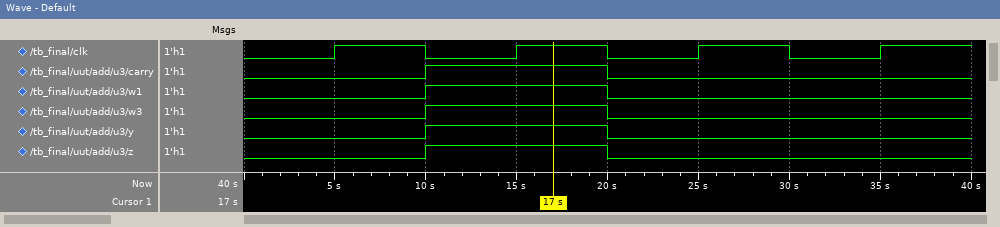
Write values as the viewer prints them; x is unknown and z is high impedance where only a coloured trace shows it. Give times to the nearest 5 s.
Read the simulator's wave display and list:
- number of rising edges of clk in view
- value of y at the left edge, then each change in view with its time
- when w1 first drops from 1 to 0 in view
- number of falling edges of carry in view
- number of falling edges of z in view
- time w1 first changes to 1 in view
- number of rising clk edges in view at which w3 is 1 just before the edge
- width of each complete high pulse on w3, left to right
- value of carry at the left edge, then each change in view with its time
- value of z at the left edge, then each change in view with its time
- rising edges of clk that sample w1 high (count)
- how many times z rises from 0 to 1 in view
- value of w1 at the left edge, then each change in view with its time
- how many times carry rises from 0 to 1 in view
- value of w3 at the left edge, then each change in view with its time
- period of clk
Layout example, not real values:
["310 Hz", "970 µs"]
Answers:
["4", "0, 1 at 10 s, 0 at 20 s", "20 s", "1", "1", "10 s", "1", "10 s", "0, 1 at 10 s, 0 at 20 s", "0, 1 at 10 s, 0 at 20 s", "1", "1", "0, 1 at 10 s, 0 at 20 s", "1", "0, 1 at 10 s, 0 at 20 s", "10 s"]
